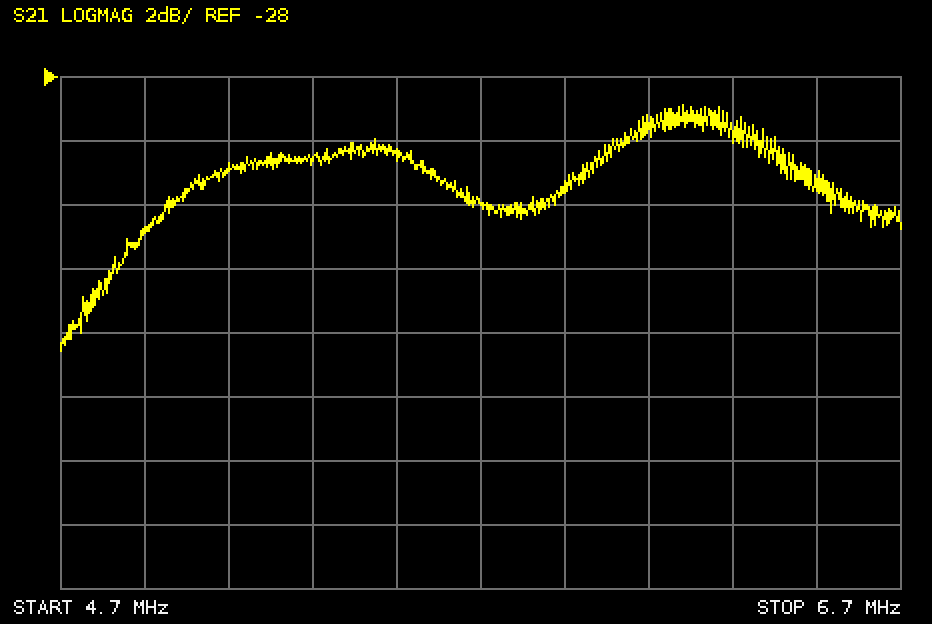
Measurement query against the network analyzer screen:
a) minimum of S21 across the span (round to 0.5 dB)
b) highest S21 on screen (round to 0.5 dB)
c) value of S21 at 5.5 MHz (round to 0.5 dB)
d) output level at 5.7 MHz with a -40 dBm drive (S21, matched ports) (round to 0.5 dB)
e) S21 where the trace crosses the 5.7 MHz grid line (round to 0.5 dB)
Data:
-36.5 dB
-29.0 dB
-30.5 dB
-72.0 dBm
-32.0 dB
